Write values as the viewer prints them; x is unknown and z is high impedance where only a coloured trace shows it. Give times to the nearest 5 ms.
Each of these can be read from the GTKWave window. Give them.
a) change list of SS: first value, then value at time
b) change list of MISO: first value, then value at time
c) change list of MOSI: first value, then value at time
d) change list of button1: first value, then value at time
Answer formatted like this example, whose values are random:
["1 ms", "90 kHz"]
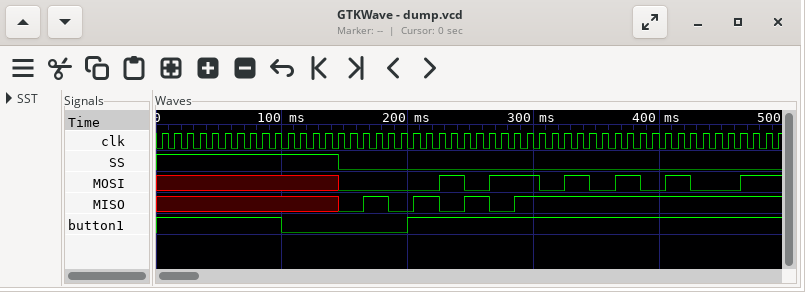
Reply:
["1, 0 at 145 ms", "x, 0 at 145 ms, 1 at 165 ms, 0 at 185 ms, 1 at 205 ms, 0 at 225 ms, 1 at 245 ms, 0 at 265 ms, 1 at 285 ms", "x, 0 at 145 ms, 1 at 225 ms, 0 at 245 ms, 1 at 265 ms, 0 at 305 ms, 1 at 325 ms, 0 at 345 ms, 1 at 365 ms, 0 at 385 ms, 1 at 405 ms, 0 at 425 ms, 1 at 465 ms", "1, 0 at 100 ms, 1 at 200 ms"]
